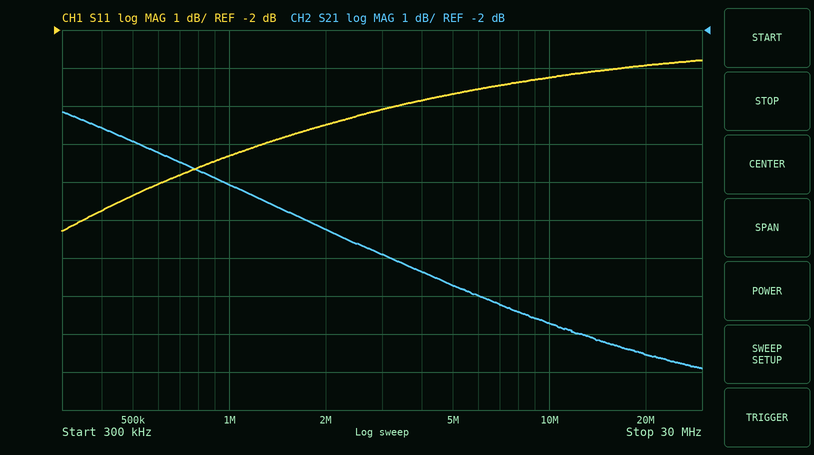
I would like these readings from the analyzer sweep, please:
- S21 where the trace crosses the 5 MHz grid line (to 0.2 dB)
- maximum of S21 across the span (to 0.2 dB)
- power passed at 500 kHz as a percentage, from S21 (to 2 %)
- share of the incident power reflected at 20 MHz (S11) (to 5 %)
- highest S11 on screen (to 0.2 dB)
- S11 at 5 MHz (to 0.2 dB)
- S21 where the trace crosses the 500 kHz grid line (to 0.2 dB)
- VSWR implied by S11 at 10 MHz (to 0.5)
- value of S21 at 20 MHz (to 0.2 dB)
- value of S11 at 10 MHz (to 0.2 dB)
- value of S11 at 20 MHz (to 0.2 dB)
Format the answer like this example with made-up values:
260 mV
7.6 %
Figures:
-8.8 dB
-4.2 dB
32 %
50 %
-2.8 dB
-3.6 dB
-5.0 dB
5.5
-10.6 dB
-3.2 dB
-3.0 dB
